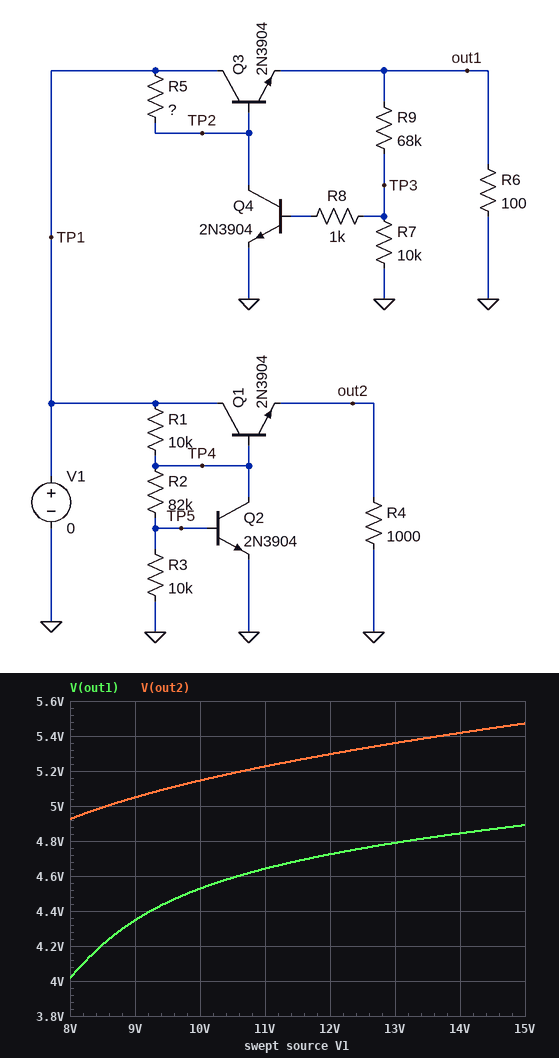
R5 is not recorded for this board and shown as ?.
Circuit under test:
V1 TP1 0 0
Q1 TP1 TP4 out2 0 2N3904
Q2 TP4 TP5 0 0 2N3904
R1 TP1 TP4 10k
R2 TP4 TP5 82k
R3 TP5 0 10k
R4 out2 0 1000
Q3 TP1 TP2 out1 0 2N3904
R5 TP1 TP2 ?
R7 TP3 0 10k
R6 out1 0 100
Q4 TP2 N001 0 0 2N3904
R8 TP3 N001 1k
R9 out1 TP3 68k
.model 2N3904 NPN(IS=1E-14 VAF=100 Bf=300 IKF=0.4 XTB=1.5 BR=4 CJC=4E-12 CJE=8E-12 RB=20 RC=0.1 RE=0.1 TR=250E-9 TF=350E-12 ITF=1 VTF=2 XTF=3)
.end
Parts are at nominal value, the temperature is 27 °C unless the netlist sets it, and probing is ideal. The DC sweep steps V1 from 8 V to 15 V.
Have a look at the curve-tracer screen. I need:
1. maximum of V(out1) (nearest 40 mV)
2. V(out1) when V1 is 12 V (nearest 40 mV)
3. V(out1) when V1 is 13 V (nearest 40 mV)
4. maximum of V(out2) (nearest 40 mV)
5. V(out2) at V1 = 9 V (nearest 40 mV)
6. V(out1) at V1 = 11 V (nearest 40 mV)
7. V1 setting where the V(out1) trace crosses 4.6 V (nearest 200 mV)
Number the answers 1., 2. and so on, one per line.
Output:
1. 4.88 V
2. 4.72 V
3. 4.80 V
4. 5.48 V
5. 5.04 V
6. 4.64 V
7. 10.6 V
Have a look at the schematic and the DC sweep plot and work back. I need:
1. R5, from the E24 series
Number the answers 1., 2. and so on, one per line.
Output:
1. 22 kΩ
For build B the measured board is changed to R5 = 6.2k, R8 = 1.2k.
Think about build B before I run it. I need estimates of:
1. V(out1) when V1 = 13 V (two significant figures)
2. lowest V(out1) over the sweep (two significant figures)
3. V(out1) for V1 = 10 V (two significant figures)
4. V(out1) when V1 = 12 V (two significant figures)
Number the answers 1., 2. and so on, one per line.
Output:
1. 5.3 V
2. 4.8 V
3. 5.1 V
4. 5.2 V
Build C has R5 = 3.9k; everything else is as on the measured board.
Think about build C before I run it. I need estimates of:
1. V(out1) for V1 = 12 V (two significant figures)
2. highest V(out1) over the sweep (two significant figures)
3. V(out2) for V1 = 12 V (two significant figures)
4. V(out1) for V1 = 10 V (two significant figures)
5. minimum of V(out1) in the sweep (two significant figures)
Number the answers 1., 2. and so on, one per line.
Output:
1. 5.5 V
2. 5.7 V
3. 5.3 V
4. 5.3 V
5. 5.0 V
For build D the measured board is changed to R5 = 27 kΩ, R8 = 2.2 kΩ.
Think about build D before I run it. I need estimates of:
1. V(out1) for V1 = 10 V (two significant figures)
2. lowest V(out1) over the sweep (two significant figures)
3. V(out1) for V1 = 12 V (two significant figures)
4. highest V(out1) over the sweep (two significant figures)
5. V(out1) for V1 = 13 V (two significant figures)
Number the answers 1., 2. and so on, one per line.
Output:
1. 4.4 V
2. 3.7 V
3. 4.6 V
4. 4.8 V
5. 4.7 V
